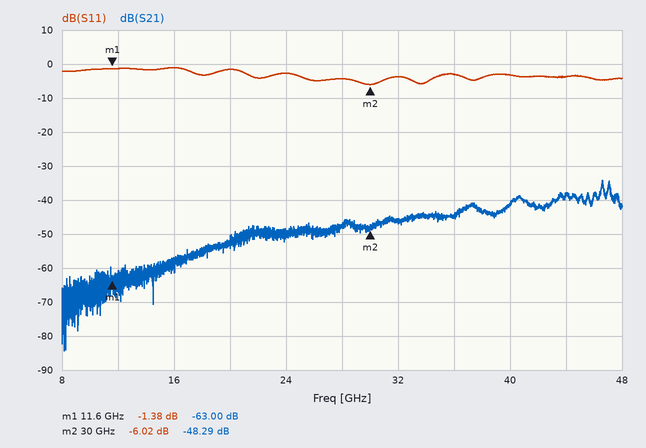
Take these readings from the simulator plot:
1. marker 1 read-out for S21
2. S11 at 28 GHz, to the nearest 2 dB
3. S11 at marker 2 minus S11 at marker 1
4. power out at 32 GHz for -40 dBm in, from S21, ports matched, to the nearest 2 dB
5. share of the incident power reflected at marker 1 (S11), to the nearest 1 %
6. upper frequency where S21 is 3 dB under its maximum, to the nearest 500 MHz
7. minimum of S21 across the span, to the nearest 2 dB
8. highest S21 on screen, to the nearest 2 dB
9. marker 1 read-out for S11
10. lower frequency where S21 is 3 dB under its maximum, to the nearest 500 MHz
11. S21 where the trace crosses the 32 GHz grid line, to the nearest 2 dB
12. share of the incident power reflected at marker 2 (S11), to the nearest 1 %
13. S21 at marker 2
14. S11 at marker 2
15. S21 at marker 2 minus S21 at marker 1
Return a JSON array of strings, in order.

["-63.00 dB", "-4 dB", "-4.64 dB", "-86 dBm", "73 %", "46.5 GHz", "-84 dB", "-34 dB", "-1.38 dB", "46.5 GHz", "-46 dB", "25 %", "-48.29 dB", "-6.02 dB", "14.71 dB"]
